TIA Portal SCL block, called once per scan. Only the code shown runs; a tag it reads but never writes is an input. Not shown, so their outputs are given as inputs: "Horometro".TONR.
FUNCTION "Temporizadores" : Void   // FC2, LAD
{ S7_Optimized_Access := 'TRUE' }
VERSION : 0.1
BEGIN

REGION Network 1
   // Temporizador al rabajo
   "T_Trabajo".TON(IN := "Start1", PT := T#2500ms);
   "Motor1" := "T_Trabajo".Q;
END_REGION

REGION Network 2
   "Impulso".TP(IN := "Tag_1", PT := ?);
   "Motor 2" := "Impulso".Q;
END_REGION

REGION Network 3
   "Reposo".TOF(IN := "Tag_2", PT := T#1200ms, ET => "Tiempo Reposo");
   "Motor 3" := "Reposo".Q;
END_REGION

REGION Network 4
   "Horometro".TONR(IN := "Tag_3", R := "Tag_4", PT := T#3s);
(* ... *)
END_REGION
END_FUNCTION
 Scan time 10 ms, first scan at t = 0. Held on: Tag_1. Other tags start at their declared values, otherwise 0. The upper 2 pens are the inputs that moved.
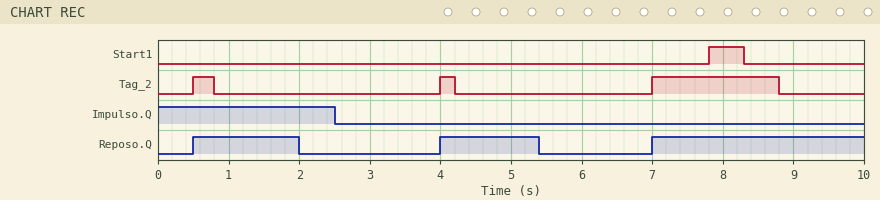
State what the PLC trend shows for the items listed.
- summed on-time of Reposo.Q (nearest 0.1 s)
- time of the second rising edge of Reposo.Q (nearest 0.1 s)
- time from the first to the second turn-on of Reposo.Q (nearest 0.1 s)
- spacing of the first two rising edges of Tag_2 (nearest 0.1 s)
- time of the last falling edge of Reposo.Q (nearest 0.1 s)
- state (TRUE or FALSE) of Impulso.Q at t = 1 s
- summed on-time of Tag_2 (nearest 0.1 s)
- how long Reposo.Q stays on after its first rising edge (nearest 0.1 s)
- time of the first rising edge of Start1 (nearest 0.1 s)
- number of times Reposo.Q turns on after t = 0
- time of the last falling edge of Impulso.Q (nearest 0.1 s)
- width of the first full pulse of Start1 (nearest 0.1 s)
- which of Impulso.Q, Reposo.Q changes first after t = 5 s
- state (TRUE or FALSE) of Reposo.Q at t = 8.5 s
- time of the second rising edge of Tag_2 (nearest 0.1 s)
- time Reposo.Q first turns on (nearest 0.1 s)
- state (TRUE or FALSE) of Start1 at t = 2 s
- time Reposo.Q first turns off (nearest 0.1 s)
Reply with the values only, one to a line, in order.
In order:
5.9 s
4.0 s
3.5 s
3.5 s
5.4 s
TRUE
2.3 s
1.5 s
7.8 s
3
2.5 s
0.5 s
Reposo.Q
TRUE
4.0 s
0.5 s
FALSE
2.0 s
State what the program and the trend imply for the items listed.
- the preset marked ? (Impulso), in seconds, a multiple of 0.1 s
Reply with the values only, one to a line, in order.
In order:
2.5 s
